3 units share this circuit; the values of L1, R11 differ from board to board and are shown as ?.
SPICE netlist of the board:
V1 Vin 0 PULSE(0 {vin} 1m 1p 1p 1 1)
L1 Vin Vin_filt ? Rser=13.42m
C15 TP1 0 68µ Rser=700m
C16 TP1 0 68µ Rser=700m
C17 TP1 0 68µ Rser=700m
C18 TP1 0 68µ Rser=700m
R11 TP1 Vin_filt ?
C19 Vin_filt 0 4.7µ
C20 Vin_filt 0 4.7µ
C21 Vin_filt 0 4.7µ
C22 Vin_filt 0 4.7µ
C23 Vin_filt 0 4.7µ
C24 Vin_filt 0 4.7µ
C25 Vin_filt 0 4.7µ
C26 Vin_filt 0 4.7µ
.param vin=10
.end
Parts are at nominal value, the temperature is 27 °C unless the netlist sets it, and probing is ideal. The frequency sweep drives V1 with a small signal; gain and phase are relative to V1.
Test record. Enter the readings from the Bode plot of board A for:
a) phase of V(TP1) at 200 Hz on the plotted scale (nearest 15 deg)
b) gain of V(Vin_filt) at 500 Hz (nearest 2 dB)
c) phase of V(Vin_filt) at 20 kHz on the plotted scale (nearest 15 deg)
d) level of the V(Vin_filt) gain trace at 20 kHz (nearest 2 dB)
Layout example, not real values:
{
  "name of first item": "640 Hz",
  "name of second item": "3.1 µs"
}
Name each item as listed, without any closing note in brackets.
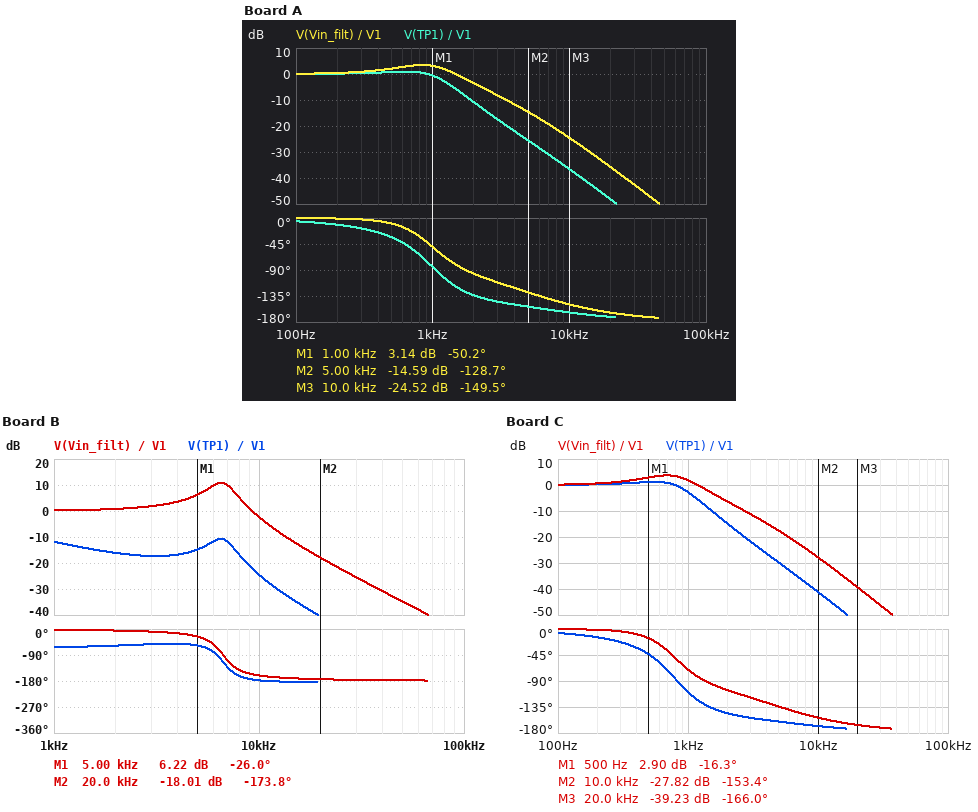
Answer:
{
  "phase of V(TP1) at 200 Hz on the plotted scale": "-15 deg",
  "gain of V(Vin_filt) at 500 Hz": "2 dB",
  "phase of V(Vin_filt) at 20 kHz on the plotted scale": "-165 deg",
  "level of the V(Vin_filt) gain trace at 20 kHz": "-36 dB"
}
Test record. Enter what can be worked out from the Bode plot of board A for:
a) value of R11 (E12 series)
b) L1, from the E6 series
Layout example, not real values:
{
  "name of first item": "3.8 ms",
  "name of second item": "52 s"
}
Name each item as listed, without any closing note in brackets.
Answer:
{
  "value of R11": "0.56 Ω",
  "L1, from the E6 series": "100 µH"
}
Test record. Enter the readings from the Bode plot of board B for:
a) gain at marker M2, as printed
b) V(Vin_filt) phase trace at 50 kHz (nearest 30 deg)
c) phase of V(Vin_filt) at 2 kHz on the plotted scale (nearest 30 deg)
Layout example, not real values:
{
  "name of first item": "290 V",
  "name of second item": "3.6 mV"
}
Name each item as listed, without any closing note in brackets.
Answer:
{
  "gain at marker M2, as printed": "-18.01 dB",
  "V(Vin_filt) phase trace at 50 kHz": "-180 deg",
  "phase of V(Vin_filt) at 2 kHz on the plotted scale": "0 deg"
}
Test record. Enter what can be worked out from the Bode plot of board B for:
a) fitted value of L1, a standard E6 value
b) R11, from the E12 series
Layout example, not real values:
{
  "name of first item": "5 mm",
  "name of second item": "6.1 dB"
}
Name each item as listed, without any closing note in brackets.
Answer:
{
  "fitted value of L1, a standard E6 value": "15 µH",
  "R11, from the E12 series": "2.2 Ω"
}
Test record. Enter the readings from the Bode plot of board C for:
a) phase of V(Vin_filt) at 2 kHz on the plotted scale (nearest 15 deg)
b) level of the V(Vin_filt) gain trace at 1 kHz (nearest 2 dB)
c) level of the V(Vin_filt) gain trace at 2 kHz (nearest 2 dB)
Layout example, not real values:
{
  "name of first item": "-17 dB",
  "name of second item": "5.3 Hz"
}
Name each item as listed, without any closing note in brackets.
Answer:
{
  "phase of V(Vin_filt) at 2 kHz on the plotted scale": "-105 deg",
  "level of the V(Vin_filt) gain trace at 1 kHz": "2 dB",
  "level of the V(Vin_filt) gain trace at 2 kHz": "-6 dB"
}
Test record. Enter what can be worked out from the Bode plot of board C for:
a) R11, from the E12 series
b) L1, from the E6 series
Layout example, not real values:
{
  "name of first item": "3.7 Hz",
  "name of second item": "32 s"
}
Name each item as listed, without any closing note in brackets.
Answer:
{
  "R11, from the E12 series": "0.68 Ω",
  "L1, from the E6 series": "150 µH"
}
